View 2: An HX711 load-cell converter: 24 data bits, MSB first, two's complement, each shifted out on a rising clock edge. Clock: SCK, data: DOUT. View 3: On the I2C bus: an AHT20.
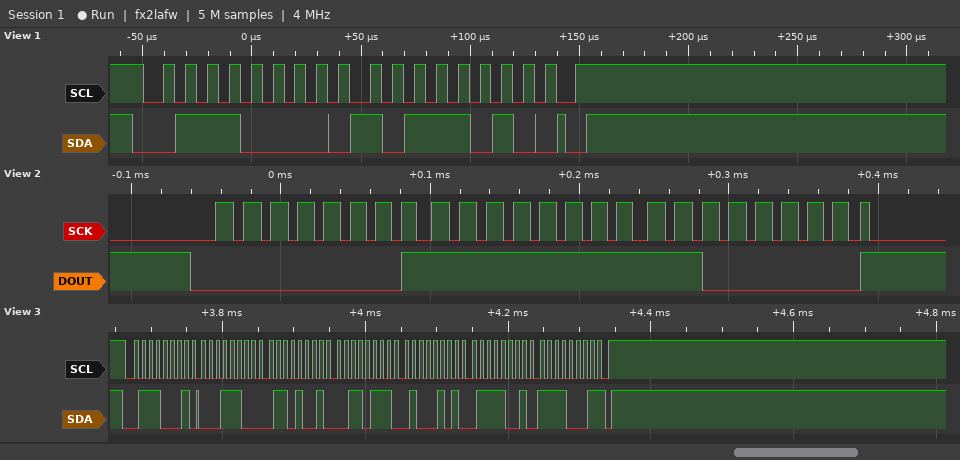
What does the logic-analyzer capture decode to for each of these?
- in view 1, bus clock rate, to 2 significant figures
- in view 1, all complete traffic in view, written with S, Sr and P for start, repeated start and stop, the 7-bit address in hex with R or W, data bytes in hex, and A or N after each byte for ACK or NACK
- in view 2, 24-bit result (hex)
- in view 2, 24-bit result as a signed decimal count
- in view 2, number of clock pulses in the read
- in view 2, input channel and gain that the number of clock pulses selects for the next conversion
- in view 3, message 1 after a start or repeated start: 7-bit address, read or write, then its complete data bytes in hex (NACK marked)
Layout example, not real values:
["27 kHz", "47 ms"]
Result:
["100 kHz", "S 38W A BA A P", "0x01FFC0", "131008", "25", "channel A, gain 128", "0x38 read: 1C 69 37 45 79 F1 NACK"]
